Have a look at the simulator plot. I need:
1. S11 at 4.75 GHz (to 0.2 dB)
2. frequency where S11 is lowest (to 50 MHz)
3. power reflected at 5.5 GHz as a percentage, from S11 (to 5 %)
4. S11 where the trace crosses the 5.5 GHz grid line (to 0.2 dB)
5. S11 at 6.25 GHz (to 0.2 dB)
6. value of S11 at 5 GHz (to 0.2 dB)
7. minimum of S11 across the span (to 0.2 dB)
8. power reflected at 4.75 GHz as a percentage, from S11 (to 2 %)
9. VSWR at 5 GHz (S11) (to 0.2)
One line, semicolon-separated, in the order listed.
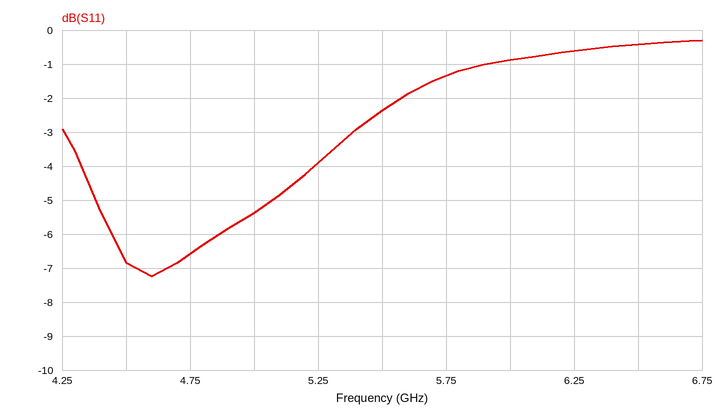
-6.6 dB; 4.60 GHz; 60 %; -2.4 dB; -0.6 dB; -5.4 dB; -7.2 dB; 22 %; 3.4
